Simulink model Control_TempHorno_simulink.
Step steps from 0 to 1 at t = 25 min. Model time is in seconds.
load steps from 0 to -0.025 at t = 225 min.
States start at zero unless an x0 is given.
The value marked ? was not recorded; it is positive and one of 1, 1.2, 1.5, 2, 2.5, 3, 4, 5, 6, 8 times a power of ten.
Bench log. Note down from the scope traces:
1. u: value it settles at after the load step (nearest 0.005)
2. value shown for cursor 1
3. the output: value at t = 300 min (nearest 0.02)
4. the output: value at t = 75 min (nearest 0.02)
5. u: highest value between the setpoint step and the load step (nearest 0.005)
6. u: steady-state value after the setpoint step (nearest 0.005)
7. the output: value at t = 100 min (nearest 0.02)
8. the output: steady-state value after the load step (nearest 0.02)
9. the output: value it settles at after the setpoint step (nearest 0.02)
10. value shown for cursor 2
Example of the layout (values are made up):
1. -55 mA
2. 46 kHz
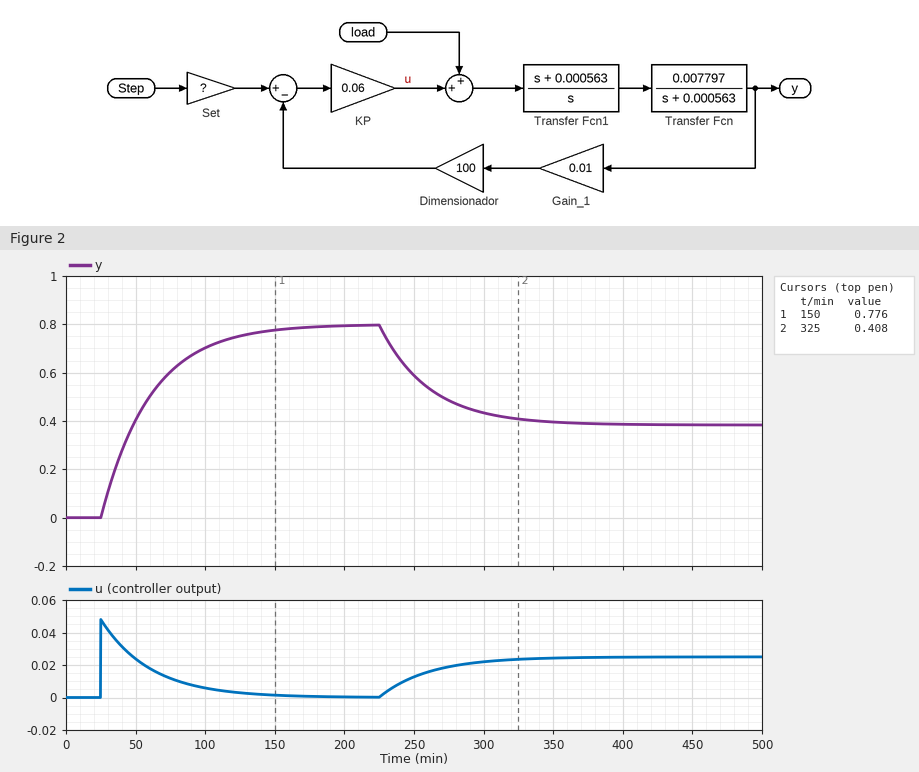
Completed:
1. 0.025
2. 0.776
3. 0.44
4. 0.60
5. 0.050
6. 0.000
7. 0.70
8. 0.38
9. 0.80
10. 0.408
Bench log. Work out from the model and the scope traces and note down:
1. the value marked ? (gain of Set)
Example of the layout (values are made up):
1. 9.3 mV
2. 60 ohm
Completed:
1. 0.8
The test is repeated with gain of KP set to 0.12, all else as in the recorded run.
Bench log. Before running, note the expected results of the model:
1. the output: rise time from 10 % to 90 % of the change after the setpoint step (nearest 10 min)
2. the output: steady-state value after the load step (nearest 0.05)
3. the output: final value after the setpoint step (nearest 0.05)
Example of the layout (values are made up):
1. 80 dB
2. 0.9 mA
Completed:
1. 40 min
2. 0.60
3. 0.80
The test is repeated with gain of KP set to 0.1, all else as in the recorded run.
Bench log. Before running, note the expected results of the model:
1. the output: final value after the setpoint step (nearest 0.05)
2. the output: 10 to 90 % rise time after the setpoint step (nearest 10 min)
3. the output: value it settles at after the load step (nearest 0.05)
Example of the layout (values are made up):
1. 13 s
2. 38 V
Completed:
1. 0.80
2. 50 min
3. 0.55
